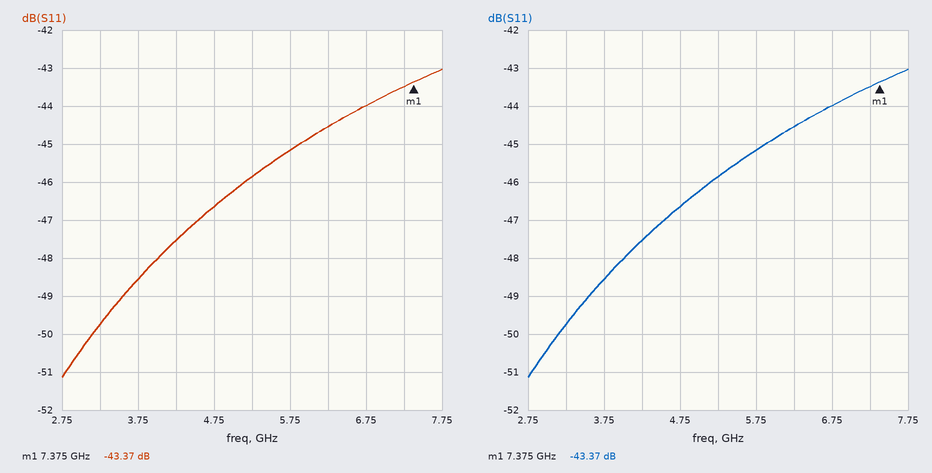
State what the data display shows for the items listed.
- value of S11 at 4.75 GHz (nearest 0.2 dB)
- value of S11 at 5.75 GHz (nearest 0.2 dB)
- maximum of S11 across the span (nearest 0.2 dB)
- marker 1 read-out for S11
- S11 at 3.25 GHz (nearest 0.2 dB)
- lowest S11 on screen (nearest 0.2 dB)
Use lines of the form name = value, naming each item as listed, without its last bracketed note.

value of S11 at 4.75 GHz = -46.6 dB
value of S11 at 5.75 GHz = -45.2 dB
maximum of S11 across the span = -43.0 dB
marker 1 read-out for S11 = -43.37 dB
S11 at 3.25 GHz = -49.8 dB
lowest S11 on screen = -51.2 dB
